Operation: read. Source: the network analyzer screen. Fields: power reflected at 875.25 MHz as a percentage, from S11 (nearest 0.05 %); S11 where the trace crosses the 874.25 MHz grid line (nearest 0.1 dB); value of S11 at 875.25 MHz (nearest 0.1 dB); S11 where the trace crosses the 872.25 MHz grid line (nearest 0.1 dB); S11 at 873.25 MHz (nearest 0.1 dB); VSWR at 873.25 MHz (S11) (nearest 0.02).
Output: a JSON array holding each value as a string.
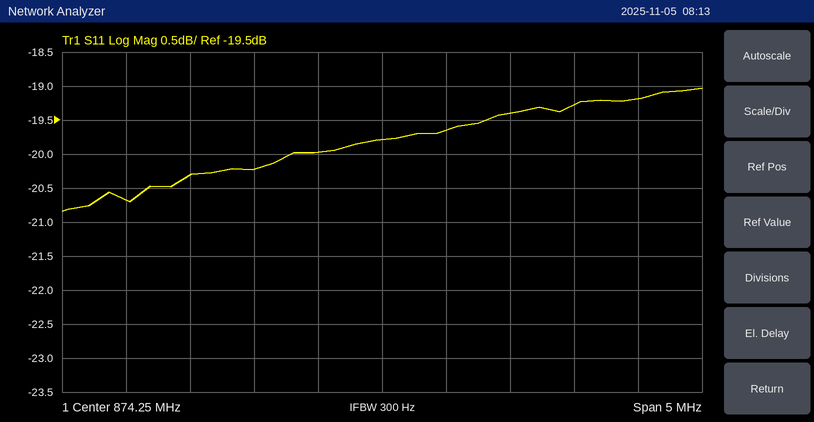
["1.15 %", "-19.8 dB", "-19.4 dB", "-20.7 dB", "-20.2 dB", "1.22"]
